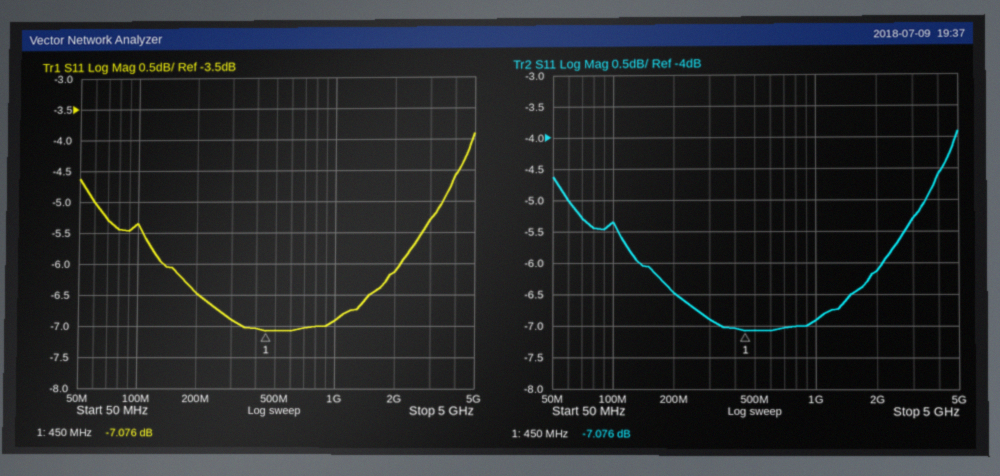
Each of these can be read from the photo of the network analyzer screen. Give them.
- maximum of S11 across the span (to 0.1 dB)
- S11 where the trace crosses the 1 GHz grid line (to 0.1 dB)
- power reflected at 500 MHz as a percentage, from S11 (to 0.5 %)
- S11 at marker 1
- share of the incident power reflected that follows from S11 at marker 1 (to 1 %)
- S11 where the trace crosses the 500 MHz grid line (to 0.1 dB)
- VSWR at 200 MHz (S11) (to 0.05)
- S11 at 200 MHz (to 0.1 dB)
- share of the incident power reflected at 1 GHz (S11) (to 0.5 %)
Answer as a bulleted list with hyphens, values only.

- -3.9 dB
- -6.9 dB
- 19.5 %
- -7.076 dB
- 20 %
- -7.1 dB
- 2.80
- -6.5 dB
- 20.5 %
